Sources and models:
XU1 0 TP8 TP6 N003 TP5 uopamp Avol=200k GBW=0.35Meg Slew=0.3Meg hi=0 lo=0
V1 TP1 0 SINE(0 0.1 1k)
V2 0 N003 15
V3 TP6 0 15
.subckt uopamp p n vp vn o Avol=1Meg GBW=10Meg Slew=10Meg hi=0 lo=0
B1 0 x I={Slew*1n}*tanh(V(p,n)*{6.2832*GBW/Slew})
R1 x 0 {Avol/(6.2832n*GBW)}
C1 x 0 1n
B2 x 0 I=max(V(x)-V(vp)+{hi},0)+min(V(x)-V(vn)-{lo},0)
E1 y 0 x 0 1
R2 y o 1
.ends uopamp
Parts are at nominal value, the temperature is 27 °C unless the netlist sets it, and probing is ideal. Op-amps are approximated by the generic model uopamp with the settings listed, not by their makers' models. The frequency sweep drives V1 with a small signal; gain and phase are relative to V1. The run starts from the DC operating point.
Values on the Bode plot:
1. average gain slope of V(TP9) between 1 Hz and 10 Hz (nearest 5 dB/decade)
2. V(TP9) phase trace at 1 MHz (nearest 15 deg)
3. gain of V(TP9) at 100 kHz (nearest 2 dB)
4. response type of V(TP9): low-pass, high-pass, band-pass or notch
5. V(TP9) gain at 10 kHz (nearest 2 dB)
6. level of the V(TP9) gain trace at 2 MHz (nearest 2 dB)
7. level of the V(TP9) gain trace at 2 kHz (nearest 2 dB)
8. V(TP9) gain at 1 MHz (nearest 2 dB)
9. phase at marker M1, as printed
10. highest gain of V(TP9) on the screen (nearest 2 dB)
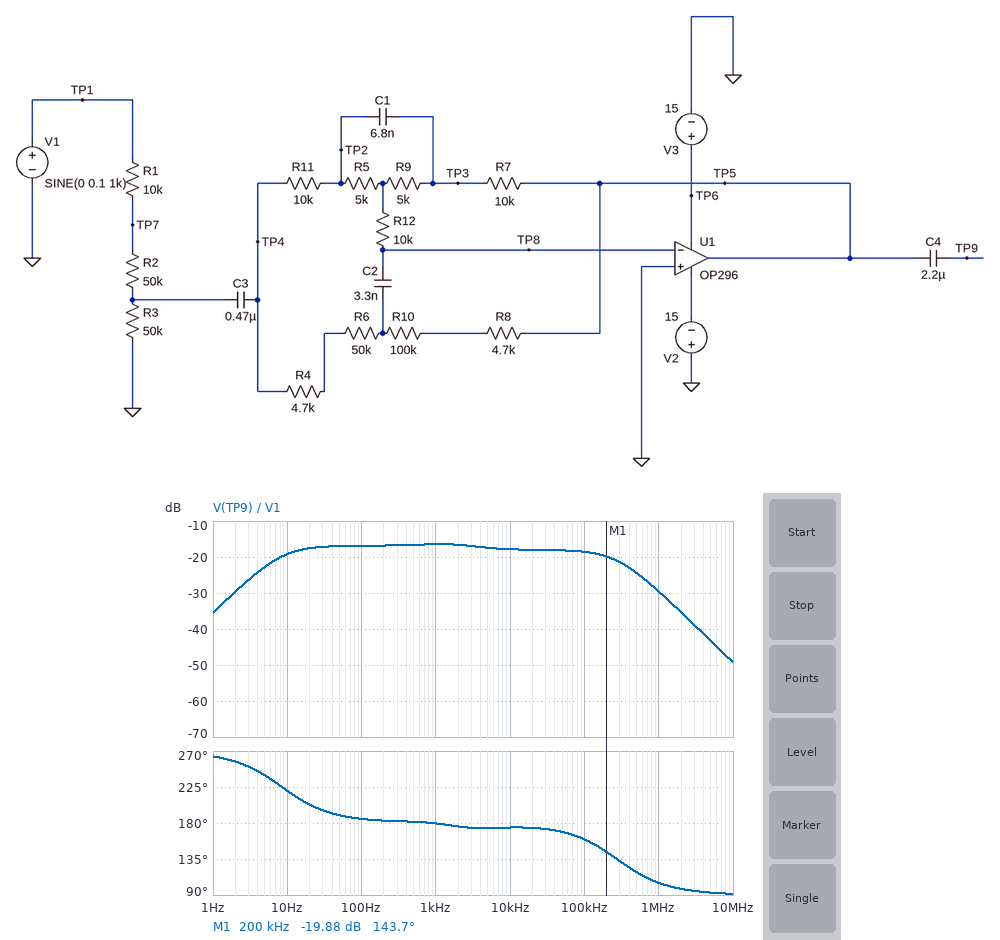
15 dB/decade
105 deg
-18 dB
band-pass
-18 dB
-36 dB
-16 dB
-30 dB
143.7 deg
-16 dB
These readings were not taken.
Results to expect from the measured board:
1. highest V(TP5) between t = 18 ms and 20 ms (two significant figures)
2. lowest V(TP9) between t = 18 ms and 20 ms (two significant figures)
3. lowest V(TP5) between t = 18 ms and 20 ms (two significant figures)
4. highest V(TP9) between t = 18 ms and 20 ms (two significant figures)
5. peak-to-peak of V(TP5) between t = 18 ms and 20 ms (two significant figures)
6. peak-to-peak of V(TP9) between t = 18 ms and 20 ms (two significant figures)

15 mV
-15 mV
-15 mV
15 mV
30 mV
30 mV
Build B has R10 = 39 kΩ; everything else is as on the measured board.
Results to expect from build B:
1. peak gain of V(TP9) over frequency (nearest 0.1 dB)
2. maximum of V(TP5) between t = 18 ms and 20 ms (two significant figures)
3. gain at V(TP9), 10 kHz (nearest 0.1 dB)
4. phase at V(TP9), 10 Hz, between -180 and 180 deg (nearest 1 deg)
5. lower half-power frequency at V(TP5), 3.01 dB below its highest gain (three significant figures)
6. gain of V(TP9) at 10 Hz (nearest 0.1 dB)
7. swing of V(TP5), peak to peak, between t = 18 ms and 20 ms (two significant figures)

-17.4 dB
13 mV
-19.8 dB
-139 deg
8.68 Hz
-19.9 dB
26 mV
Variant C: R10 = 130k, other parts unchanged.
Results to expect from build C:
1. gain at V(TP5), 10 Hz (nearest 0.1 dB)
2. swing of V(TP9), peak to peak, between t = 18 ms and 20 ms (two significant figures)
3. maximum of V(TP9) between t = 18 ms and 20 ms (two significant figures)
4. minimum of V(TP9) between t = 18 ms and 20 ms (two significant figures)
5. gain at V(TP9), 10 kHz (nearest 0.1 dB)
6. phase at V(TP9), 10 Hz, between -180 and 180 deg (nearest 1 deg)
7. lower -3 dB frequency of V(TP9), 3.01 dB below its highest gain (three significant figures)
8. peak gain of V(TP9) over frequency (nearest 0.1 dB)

-19.0 dB
31 mV
16 mV
-16 mV
-17.5 dB
-140 deg
9.81 Hz
-16.1 dB
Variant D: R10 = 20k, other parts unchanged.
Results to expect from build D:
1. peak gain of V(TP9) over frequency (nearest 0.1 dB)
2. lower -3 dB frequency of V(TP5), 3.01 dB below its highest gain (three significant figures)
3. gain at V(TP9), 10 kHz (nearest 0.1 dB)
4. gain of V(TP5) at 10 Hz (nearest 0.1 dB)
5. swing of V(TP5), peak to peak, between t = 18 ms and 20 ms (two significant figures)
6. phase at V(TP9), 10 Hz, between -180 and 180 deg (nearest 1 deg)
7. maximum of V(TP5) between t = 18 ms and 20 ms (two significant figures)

-17.8 dB
8.79 Hz
-21.9 dB
-20.3 dB
23 mV
-139 deg
12 mV
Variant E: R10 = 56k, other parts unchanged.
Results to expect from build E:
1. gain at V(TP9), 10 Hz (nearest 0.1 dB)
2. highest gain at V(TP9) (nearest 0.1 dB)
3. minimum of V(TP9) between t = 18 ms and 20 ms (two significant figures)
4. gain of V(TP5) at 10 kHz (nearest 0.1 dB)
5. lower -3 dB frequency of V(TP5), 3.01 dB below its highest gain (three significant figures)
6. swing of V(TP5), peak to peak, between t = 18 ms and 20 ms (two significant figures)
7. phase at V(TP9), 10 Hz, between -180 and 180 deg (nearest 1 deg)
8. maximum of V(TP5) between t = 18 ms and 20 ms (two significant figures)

-19.6 dB
-17.2 dB
-14 mV
-18.9 dB
8.63 Hz
27 mV
-139 deg
14 mV
